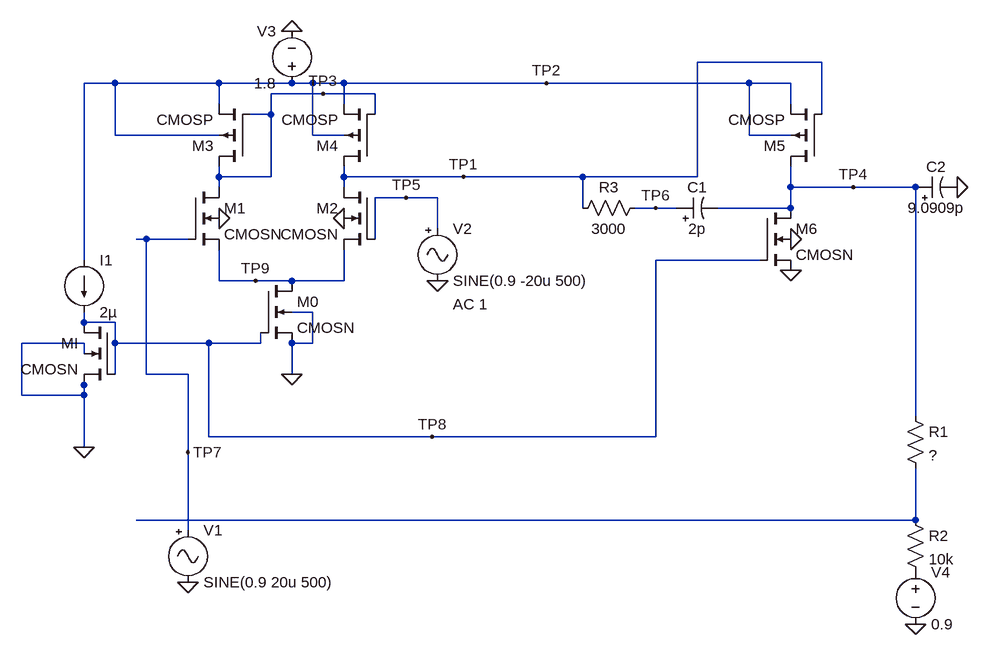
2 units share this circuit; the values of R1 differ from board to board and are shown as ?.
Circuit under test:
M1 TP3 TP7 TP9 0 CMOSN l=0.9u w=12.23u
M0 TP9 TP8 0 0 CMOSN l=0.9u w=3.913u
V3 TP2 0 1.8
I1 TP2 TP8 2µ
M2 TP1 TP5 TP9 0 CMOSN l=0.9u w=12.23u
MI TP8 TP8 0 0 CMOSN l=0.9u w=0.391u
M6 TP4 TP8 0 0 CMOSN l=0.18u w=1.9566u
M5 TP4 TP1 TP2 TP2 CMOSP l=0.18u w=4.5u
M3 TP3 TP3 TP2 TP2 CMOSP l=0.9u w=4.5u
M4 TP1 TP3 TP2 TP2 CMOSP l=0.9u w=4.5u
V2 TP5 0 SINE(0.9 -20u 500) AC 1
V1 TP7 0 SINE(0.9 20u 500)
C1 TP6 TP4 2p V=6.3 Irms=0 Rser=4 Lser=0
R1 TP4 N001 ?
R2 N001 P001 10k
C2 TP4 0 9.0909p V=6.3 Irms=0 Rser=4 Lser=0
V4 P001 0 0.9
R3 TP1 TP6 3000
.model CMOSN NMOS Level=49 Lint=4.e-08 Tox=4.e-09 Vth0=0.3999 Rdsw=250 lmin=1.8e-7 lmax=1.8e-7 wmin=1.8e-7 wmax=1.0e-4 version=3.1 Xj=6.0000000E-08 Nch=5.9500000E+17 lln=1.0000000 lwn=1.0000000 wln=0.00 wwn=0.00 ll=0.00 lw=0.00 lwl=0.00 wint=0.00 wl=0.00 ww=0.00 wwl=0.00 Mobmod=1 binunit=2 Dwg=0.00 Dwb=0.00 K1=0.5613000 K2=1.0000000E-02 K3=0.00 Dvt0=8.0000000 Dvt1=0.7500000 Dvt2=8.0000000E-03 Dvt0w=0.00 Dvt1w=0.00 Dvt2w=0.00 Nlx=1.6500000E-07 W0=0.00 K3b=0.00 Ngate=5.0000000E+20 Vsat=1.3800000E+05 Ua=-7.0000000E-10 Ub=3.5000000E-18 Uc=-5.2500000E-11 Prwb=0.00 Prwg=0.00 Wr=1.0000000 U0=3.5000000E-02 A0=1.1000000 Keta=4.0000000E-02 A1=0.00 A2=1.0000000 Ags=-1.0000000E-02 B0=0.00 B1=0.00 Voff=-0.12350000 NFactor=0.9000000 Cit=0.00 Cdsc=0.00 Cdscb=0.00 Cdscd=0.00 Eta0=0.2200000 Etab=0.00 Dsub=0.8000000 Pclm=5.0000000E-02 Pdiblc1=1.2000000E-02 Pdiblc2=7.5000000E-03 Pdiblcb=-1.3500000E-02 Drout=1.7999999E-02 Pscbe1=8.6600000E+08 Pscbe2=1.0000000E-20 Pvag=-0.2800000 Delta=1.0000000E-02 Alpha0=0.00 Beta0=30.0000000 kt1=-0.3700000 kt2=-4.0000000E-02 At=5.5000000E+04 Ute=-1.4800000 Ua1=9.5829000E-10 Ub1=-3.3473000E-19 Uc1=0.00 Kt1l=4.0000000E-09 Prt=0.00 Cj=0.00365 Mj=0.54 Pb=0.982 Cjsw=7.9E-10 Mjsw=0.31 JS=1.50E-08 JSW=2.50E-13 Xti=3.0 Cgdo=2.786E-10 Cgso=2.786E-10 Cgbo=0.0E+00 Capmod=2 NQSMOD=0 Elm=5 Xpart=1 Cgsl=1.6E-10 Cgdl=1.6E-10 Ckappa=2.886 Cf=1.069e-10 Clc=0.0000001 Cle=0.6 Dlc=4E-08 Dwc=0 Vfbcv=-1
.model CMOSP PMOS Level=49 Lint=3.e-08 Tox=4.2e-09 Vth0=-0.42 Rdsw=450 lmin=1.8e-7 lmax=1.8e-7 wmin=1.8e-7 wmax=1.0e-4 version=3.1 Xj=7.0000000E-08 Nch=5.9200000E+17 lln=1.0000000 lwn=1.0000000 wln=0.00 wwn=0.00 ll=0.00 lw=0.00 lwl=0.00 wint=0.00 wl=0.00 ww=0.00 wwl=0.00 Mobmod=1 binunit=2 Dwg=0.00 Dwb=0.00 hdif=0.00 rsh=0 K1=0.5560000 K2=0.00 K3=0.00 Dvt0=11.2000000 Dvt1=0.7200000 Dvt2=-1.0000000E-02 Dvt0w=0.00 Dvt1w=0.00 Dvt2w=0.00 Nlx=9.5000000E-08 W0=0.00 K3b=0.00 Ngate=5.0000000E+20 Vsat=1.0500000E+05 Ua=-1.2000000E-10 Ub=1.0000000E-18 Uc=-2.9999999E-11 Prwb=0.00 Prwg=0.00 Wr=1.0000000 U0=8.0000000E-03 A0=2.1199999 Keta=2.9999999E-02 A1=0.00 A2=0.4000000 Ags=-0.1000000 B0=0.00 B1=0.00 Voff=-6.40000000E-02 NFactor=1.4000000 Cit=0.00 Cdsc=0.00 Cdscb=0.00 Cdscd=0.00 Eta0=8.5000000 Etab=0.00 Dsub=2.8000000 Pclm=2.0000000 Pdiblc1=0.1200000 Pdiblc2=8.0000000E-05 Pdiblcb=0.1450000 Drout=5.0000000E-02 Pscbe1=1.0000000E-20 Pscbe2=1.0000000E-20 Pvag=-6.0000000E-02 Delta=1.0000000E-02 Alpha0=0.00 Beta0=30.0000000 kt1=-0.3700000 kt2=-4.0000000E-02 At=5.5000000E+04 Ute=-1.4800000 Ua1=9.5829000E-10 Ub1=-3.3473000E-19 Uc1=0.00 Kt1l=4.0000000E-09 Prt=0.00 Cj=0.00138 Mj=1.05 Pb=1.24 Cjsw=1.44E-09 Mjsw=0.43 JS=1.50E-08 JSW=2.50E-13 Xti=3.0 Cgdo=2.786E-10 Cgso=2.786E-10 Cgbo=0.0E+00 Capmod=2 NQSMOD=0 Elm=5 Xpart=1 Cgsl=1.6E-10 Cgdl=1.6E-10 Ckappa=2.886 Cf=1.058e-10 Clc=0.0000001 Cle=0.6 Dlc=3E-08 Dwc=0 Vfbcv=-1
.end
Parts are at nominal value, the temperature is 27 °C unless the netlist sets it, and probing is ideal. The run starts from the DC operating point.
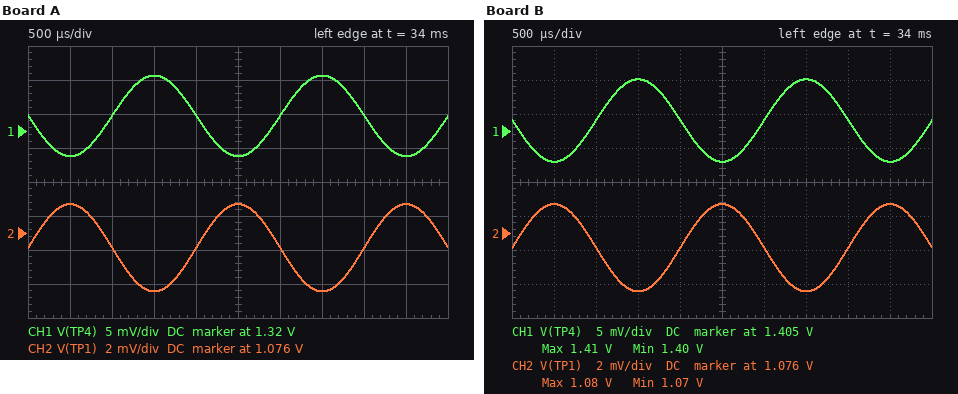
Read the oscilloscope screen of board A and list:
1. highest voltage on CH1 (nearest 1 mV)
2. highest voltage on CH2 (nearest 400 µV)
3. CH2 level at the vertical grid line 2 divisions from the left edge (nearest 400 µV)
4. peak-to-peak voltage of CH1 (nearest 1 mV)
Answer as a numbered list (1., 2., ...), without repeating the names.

1. 1.328 V
2. 1.0776 V
3. 1.0752 V
4. 12 mV
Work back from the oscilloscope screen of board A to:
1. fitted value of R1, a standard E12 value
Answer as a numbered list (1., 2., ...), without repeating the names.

1. 3.3 kΩ
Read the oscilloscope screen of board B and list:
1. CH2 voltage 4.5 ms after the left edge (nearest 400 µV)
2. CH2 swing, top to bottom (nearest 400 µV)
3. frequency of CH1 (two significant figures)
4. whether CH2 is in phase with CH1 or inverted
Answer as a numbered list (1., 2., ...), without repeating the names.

1. 1.0776 V
2. 5.2 mV
3. 500 Hz
4. inverted
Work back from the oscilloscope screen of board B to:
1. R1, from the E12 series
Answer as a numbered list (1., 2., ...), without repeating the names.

1. 27 kΩ
